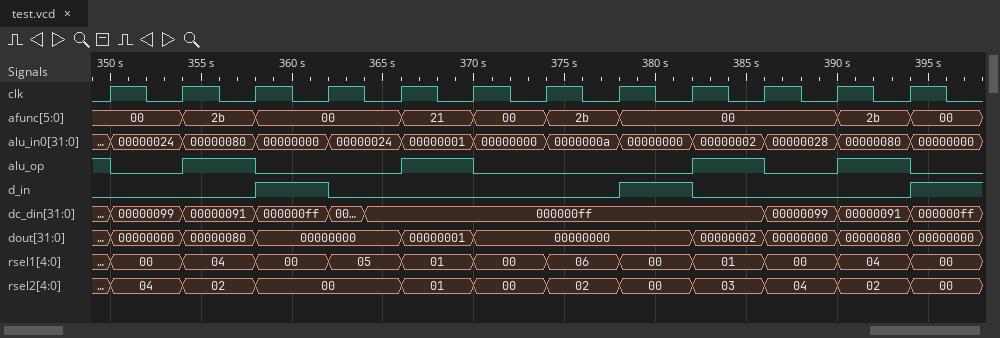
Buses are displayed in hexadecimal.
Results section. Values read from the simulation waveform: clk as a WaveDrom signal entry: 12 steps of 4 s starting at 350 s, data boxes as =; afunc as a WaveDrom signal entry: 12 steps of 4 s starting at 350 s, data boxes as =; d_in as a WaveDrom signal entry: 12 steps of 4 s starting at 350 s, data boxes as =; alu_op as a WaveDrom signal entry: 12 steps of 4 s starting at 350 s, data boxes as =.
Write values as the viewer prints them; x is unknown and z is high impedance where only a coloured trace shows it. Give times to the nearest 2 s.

{name: 'clk', wave: 'p...........'}
{name: 'afunc', wave: '===.====..==', data: '00 2b 00 21 00 2b 00 2b 00'}
{name: 'd_in', wave: '0.10...10..1'}
{name: 'alu_op', wave: '010.10..1010'}
